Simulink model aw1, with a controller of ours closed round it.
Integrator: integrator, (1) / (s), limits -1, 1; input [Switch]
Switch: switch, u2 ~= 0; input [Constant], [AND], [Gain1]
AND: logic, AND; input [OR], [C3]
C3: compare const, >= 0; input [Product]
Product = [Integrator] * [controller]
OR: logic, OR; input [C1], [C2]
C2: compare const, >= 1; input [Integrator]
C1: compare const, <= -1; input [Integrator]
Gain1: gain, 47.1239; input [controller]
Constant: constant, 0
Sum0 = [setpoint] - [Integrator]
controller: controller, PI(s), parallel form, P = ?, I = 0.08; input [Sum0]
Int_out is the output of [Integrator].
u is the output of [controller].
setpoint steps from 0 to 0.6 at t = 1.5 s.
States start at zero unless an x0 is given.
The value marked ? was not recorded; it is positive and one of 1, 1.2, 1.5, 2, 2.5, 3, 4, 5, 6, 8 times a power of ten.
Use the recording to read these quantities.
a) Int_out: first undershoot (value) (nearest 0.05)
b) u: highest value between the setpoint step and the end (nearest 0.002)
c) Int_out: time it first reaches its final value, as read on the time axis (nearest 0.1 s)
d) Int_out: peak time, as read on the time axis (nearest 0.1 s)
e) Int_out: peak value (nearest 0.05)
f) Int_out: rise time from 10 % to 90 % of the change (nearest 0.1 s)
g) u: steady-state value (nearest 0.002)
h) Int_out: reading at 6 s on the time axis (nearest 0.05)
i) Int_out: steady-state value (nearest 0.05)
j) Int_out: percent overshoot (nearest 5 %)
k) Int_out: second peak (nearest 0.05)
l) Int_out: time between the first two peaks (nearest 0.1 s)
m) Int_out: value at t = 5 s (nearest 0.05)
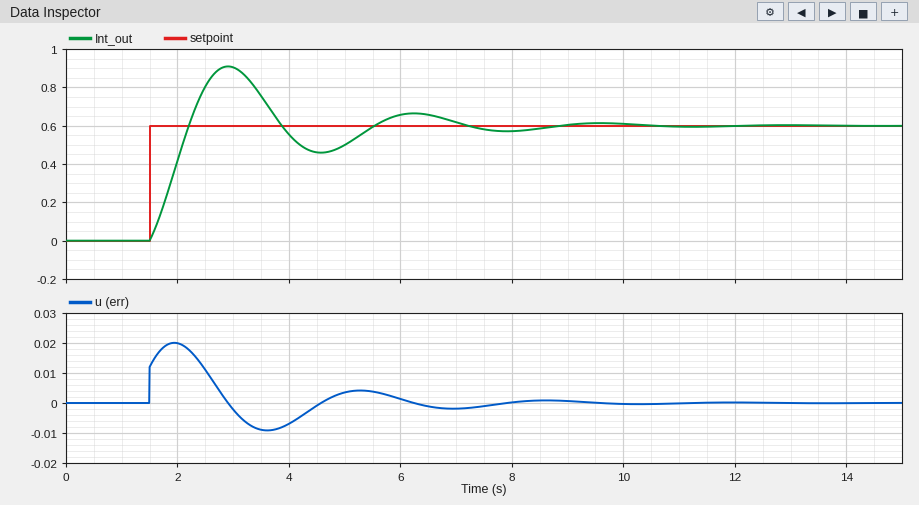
0.45
0.020
2.2 s
2.9 s
0.90
0.5 s
0.000
0.65
0.60
50 %
0.65
3.3 s
0.50
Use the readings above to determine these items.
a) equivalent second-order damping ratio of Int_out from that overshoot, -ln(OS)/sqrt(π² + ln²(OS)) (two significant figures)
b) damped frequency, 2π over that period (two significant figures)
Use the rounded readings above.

0.22
1.9 rad/s
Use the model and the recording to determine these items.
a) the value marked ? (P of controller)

0.02
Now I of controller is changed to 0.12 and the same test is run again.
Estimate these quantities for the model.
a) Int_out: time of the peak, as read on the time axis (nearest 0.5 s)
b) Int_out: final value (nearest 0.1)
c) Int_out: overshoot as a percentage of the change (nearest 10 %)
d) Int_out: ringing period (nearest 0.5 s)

2.5 s
0.6
60 %
2.5 s
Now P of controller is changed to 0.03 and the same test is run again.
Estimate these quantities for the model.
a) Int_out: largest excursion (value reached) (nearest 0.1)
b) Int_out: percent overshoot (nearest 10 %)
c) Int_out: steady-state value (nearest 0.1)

0.8
40 %
0.6
